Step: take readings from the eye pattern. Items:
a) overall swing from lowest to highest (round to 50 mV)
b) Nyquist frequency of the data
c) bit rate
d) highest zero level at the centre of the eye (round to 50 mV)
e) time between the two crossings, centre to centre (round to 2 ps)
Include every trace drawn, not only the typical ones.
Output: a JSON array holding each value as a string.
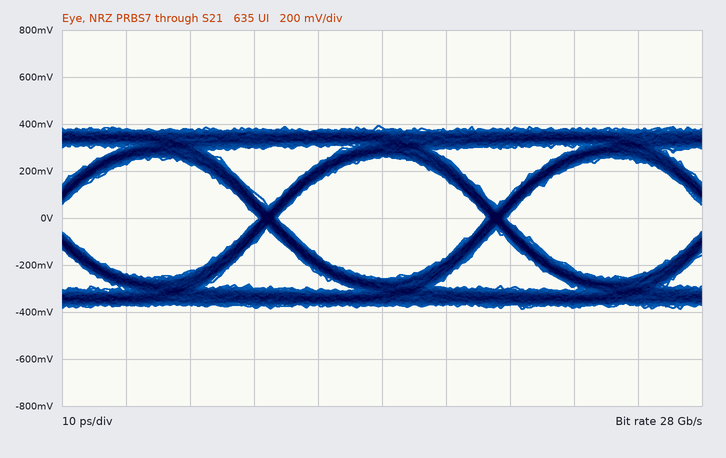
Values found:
["800 mV", "14 GHz", "28 Gb/s", "-250 mV", "36 ps"]
